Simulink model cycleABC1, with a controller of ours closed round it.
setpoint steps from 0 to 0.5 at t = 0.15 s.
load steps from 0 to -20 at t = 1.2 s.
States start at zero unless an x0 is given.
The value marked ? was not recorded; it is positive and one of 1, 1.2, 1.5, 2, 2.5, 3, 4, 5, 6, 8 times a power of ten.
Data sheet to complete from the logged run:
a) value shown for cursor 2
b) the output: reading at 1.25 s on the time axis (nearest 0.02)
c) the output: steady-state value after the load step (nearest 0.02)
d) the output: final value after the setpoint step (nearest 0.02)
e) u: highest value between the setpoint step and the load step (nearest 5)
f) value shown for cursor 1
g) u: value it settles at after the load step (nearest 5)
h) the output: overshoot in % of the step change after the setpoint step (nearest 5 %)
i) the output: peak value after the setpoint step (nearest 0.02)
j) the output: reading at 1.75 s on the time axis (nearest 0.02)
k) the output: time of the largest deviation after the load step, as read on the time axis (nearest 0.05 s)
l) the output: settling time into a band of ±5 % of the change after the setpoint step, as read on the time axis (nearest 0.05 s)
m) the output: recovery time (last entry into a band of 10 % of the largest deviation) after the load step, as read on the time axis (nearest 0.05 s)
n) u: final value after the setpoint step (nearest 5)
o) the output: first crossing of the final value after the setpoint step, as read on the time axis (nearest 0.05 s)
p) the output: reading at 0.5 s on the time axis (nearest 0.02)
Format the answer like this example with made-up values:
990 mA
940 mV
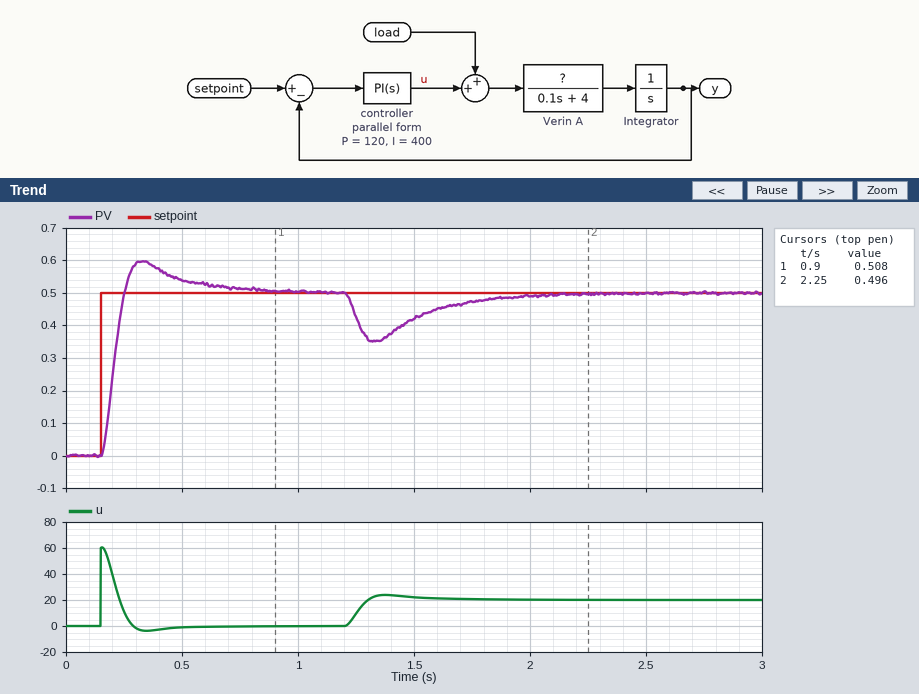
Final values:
0.496
0.42
0.50
0.50
60
0.508
20
20 %
0.60
0.48
1.35 s
0.60 s
1.90 s
0
0.25 s
0.54
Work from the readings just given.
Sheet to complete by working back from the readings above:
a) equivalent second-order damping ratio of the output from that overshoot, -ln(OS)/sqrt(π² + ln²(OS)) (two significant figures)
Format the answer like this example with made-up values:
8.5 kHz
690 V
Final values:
0.46
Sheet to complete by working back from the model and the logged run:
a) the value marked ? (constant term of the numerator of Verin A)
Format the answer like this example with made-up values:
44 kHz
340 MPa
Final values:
0.6
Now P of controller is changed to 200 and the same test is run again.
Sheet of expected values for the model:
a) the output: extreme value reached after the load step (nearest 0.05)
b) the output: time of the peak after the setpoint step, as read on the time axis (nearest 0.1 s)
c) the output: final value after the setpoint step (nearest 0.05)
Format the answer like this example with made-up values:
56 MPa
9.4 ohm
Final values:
0.40
0.3 s
0.50
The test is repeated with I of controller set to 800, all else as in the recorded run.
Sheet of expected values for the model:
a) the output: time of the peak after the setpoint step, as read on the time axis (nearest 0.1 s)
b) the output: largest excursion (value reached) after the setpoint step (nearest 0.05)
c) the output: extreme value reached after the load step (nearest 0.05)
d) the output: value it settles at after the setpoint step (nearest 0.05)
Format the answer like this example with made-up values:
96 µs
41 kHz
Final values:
0.3 s
0.65
0.35
0.50
